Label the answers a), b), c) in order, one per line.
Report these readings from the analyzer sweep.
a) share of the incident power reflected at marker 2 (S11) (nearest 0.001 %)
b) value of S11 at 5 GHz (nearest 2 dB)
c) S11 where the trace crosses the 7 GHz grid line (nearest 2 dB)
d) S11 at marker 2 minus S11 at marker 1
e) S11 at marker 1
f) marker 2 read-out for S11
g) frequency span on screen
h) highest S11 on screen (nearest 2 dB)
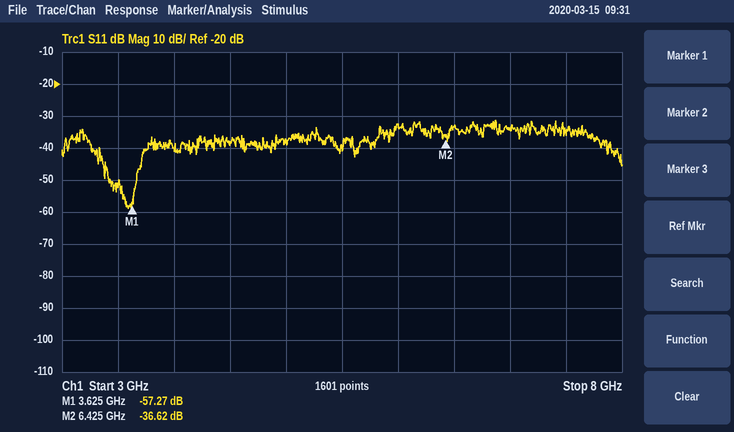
a) 0.022 %
b) -38 dB
c) -34 dB
d) 20.65 dB
e) -57.27 dB
f) -36.62 dB
g) 5 GHz
h) -32 dB
